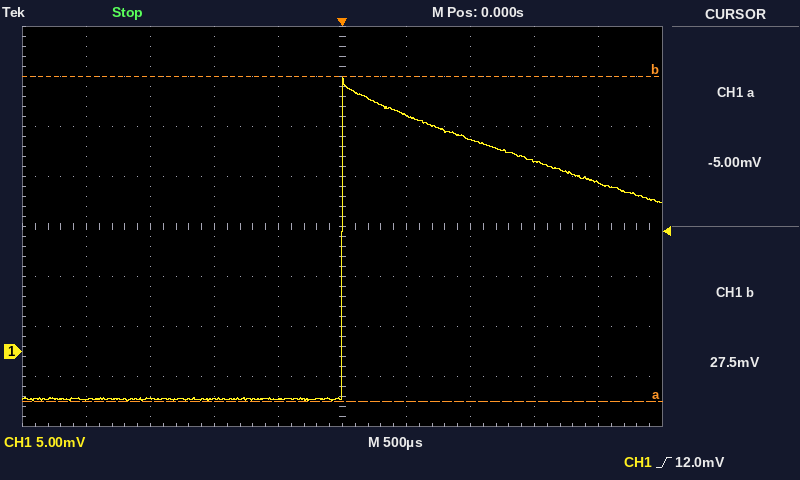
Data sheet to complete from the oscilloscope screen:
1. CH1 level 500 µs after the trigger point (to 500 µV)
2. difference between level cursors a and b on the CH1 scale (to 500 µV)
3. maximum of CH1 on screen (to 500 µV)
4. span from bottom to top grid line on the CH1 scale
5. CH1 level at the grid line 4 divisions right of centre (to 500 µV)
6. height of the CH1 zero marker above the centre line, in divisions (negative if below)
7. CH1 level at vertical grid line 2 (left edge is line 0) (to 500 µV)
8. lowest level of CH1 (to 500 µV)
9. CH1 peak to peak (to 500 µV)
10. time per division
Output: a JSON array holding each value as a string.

["23.5 mV", "32.5 mV", "27.5 mV", "40 mV", "17.0 mV", "-2.5 div", "-4.5 mV", "-5.0 mV", "32.5 mV", "500 µs"]
